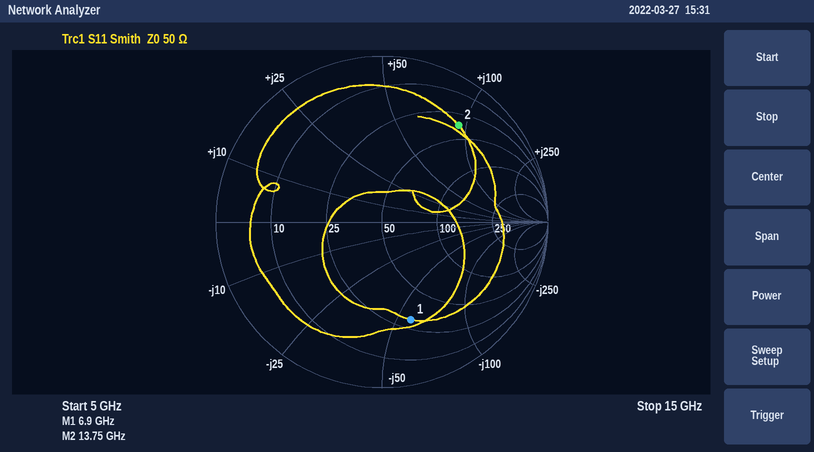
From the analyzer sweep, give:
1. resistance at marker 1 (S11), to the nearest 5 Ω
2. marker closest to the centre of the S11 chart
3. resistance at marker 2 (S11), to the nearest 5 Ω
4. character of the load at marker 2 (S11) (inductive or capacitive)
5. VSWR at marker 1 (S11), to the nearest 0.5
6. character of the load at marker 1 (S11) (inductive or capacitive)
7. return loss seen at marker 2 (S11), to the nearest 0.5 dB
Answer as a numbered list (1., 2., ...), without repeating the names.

1. 30 Ω
2. marker 1
3. 35 Ω
4. inductive
5. 4.0
6. capacitive
7. 2.5 dB
